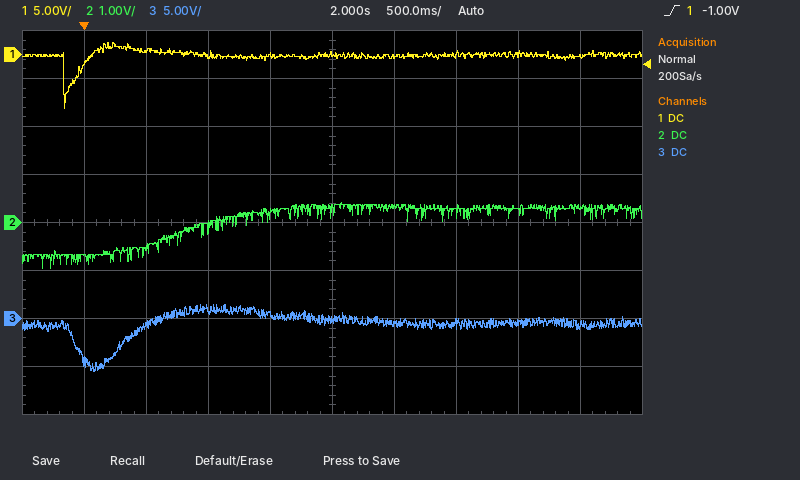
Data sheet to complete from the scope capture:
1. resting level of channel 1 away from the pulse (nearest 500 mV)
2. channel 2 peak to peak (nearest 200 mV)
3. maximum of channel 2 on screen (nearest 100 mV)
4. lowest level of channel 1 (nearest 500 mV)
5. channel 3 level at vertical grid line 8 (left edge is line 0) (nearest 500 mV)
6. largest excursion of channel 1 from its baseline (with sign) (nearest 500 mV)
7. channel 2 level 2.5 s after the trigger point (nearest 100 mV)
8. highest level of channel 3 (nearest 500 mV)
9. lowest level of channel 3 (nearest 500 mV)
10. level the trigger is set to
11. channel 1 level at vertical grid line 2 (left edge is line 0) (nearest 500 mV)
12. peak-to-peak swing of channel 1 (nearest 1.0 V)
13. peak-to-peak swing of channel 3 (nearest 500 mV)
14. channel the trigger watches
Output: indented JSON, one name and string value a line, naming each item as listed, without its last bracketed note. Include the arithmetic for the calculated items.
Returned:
{
  "resting level of channel 1 away from the pulse": "0.0 V",
  "channel 2 peak to peak": "1.4 V",
  "maximum of channel 2 on screen": "400 mV",
  "lowest level of channel 1": "-5.5 V",
  "channel 3 level at vertical grid line 8 (left edge is line 0)": "-500 mV",
  "largest excursion of channel 1 from its baseline (with sign)": "-5.5 V − (0.0 V) = -5.5 V",
  "channel 2 level 2.5 s after the trigger point": "300 mV",
  "highest level of channel 3": "1.5 V",
  "lowest level of channel 3": "-5.5 V",
  "level the trigger is set to": "-1.00 V",
  "channel 1 level at vertical grid line 2 (left edge is line 0)": "500 mV",
  "peak-to-peak swing of channel 1": "7.0 V",
  "peak-to-peak swing of channel 3": "1.5 V − (-5.5 V) = 7.0 V",
  "channel the trigger watches": "channel 1"
}
